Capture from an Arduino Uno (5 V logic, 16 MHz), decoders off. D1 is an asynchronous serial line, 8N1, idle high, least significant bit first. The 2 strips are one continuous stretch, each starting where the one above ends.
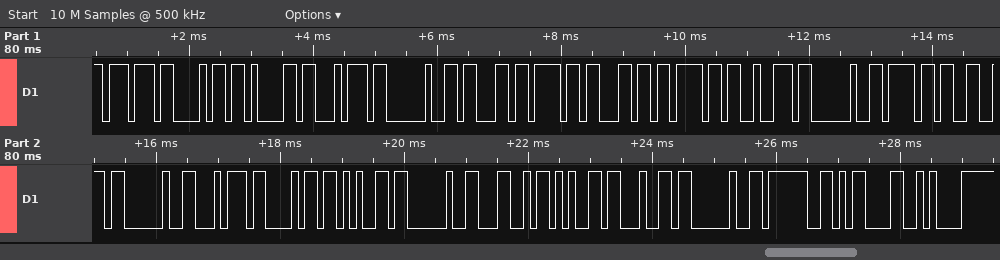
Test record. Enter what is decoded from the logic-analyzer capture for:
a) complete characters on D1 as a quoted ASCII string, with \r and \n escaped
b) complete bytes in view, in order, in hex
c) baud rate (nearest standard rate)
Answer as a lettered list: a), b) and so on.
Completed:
a) "what color of the Led ?\r\n"
b) 77 68 61 74 20 63 6F 6C 6F 72 20 6F 66 20 74 68 65 20 4C 65 64 20 3F 0D 0A
c) 9600 baud
